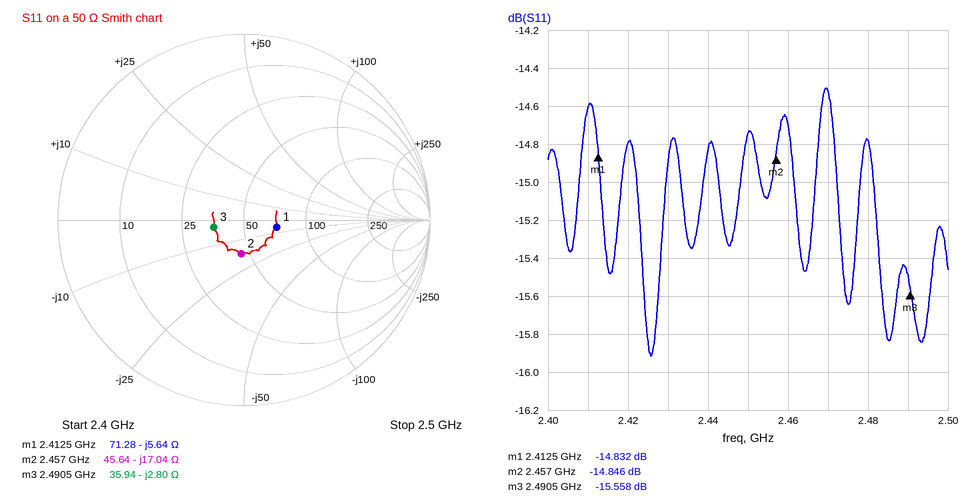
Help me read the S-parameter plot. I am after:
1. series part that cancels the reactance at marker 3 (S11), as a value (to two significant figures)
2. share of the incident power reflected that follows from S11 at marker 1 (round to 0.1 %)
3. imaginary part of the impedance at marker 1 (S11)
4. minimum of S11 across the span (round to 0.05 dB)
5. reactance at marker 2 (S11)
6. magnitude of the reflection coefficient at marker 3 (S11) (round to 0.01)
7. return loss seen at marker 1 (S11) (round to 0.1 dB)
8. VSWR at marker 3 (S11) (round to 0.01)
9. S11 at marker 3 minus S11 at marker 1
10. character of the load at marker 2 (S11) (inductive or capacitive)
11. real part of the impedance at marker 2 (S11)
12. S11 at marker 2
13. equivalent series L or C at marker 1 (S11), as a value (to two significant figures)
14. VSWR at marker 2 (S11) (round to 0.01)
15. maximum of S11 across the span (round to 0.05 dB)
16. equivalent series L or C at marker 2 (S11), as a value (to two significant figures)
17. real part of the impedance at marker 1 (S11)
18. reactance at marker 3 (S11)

180 pH
3.3 %
-5.64 Ω
-15.90 dB
-17.04 Ω
0.17
14.8 dB
1.40
-0.726 dB
capacitive
45.64 Ω
-14.846 dB
12 pF
1.44
-14.50 dB
3.8 pF
71.28 Ω
-2.80 Ω
